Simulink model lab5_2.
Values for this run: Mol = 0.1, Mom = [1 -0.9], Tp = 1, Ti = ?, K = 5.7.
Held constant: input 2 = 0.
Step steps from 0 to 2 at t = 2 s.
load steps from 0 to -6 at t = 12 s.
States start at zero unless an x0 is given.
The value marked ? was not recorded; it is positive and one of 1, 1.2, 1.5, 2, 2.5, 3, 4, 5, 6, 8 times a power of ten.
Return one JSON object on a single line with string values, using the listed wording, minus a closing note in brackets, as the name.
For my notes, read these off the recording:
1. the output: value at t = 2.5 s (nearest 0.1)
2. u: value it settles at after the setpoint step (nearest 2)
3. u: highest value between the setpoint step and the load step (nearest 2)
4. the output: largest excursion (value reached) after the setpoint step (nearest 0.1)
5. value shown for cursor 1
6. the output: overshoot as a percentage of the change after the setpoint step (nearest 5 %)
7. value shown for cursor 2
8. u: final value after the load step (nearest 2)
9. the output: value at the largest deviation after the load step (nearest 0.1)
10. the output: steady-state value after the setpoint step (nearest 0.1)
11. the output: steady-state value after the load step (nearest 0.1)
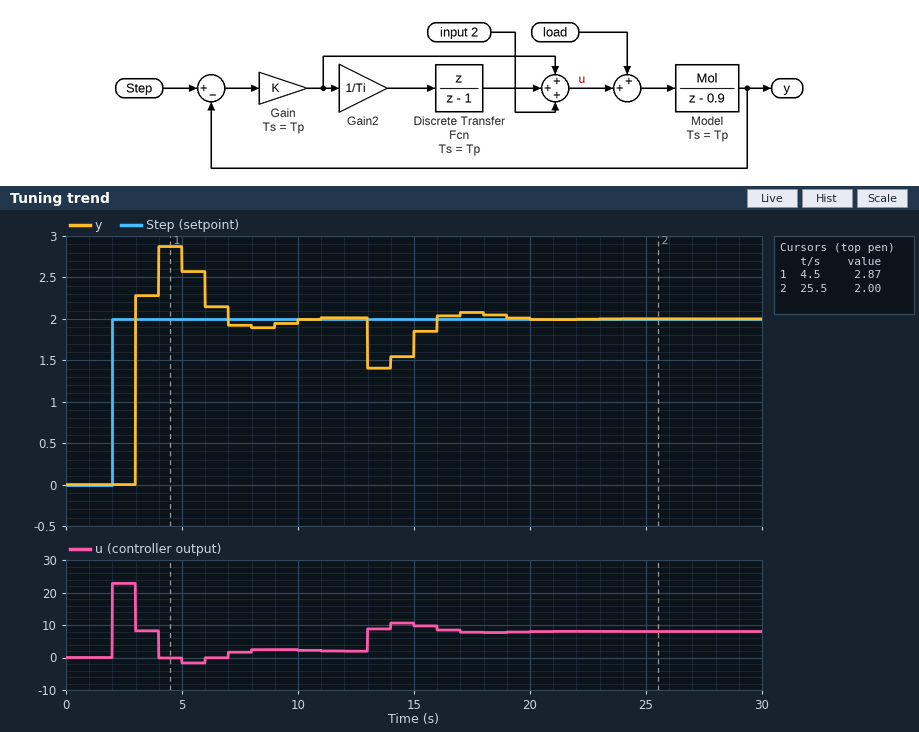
{"the output: value at t = 2.5 s": "0.0", "u: value it settles at after the setpoint step": "2", "u: highest value between the setpoint step and the load step": "22", "the output: largest excursion (value reached) after the setpoint step": "2.9", "value shown for cursor 1": "2.87", "the output: overshoot as a percentage of the change after the setpoint step": "45 %", "value shown for cursor 2": "2.00", "u: final value after the load step": "8", "the output: value at the largest deviation after the load step": "1.4", "the output: steady-state value after the setpoint step": "2.0", "the output: steady-state value after the load step": "2.0"}
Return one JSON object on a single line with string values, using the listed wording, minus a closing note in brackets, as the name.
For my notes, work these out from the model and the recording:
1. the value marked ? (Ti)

{"the value marked ?": "1"}
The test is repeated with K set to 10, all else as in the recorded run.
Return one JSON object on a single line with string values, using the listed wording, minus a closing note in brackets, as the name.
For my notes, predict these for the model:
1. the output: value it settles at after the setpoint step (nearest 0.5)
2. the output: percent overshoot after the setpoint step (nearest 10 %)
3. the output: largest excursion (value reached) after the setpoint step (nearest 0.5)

{"the output: value it settles at after the setpoint step": "2.0", "the output: percent overshoot after the setpoint step": "100 %", "the output: largest excursion (value reached) after the setpoint step": "4.0"}
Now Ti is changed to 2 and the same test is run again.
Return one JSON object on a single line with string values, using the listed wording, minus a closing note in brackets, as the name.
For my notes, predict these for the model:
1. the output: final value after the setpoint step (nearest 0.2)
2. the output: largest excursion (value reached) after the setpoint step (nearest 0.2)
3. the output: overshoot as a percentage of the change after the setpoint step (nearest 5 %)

{"the output: final value after the setpoint step": "2.0", "the output: largest excursion (value reached) after the setpoint step": "2.4", "the output: overshoot as a percentage of the change after the setpoint step": "25 %"}
